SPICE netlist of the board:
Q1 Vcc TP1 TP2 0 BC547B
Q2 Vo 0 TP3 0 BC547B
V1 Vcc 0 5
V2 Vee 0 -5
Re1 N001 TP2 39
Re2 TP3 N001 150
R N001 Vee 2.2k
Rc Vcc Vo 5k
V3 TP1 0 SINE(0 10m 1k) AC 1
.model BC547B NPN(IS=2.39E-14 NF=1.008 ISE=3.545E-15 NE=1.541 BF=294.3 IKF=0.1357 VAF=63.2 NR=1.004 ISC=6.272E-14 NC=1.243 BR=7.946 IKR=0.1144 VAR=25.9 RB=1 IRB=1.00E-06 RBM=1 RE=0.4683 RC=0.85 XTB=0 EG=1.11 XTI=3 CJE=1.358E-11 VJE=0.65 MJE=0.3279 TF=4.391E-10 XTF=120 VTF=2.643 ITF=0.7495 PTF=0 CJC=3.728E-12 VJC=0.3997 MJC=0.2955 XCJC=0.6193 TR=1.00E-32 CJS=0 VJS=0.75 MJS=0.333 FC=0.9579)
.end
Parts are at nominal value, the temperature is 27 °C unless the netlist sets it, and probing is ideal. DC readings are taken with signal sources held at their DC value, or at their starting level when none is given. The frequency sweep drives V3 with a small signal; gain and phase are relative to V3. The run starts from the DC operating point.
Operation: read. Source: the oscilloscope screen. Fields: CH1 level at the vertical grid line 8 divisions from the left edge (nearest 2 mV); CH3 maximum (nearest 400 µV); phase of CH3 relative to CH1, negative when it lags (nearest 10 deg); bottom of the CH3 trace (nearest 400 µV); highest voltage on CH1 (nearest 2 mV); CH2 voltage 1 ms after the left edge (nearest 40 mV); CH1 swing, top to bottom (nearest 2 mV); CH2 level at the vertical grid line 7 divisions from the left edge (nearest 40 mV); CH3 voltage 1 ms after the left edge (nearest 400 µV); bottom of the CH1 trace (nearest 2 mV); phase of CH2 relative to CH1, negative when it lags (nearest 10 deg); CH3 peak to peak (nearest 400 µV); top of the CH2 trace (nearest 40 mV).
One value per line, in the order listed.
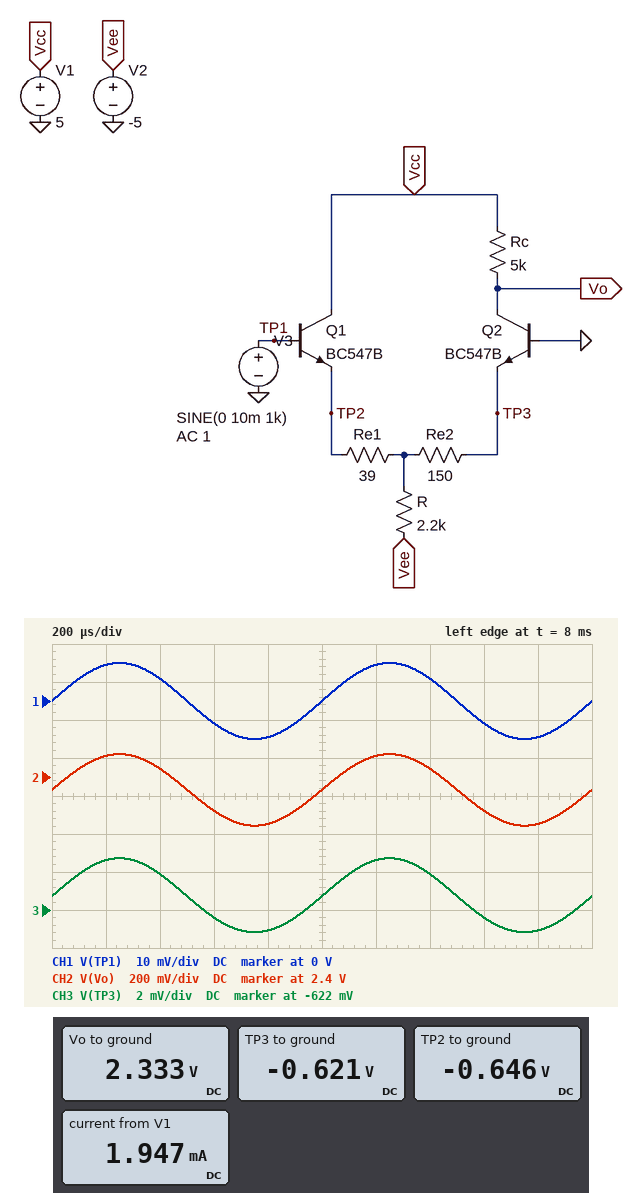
-6 mV
-619.2 mV
0 deg
-623.2 mV
10 mV
2.32 V
20 mV
2.44 V
-621.2 mV
-10 mV
0 deg
4.0 mV
2.52 V
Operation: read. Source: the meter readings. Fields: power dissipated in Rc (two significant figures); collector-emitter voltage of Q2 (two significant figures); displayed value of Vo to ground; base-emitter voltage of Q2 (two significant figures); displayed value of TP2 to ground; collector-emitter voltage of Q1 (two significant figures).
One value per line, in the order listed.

1.4 mW
3.0 V
2.333 V
620 mV
-0.646 V
5.6 V
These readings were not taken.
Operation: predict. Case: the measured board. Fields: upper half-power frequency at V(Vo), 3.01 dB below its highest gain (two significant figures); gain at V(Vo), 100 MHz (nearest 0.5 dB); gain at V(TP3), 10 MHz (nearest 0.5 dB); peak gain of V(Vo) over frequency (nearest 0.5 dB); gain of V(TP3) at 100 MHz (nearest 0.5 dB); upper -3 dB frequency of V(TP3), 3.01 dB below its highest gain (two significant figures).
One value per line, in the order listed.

15 MHz
5.5 dB
-14.5 dB
25.5 dB
-18.0 dB
86 MHz
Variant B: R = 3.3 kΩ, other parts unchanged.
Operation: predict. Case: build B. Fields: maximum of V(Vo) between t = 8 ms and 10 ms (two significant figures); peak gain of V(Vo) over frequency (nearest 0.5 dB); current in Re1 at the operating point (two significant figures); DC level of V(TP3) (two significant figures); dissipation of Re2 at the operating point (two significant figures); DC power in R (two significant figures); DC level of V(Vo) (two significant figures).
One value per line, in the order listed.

3.2 V
24.5 dB
920 µA
-610 mV
23 µW
5.7 mW
3.1 V
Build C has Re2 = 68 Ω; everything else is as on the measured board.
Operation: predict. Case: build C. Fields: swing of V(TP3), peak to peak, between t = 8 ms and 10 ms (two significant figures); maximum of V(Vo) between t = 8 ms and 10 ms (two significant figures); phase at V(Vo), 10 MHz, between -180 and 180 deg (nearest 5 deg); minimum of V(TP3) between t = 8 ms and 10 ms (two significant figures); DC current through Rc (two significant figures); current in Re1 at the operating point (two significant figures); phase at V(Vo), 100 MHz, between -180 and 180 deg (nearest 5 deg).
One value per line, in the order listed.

4.2 mV
1.3 V
-45 deg
-630 mV
790 µA
1.2 mA
-120 deg
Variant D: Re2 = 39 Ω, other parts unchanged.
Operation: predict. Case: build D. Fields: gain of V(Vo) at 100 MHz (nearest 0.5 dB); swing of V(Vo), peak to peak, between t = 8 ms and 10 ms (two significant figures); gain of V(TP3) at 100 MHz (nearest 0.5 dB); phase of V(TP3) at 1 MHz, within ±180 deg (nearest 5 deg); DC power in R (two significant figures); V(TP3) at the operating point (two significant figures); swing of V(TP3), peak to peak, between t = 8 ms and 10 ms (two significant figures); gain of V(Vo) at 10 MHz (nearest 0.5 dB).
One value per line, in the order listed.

9.5 dB
730 mV
-15.0 dB
0 deg
8.5 mW
-640 mV
4.4 mV
28.0 dB
